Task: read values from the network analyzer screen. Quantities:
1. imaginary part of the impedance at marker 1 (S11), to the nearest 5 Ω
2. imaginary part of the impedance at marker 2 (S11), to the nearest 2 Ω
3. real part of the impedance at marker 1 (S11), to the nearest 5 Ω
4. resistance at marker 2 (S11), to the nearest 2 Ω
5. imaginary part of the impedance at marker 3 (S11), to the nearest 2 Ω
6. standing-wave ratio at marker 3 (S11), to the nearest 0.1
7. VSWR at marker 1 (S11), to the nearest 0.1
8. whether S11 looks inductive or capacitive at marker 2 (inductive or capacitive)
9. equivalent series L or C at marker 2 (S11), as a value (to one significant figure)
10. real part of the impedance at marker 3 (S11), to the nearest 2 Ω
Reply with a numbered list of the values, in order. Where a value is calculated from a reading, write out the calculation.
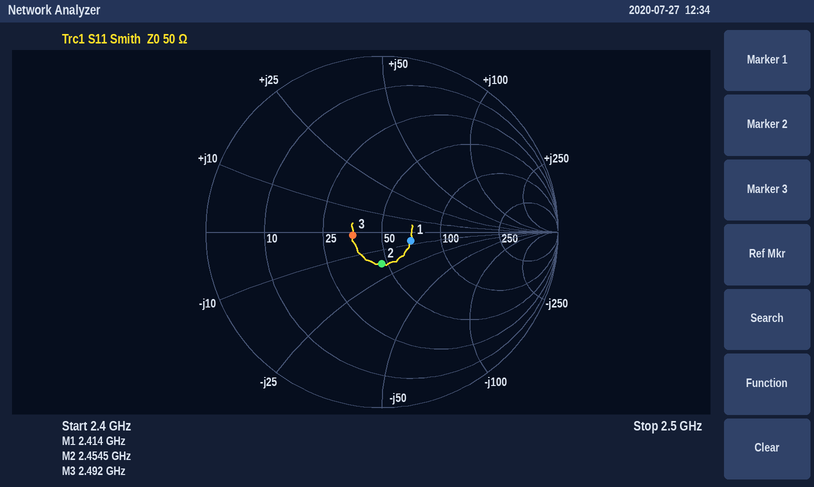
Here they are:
1. -5 Ω
2. -18 Ω
3. 70 Ω
4. 46 Ω
5. -2 Ω
6. 1.4
7. 1.4
8. capacitive
9. C = 1/(2π × 2.4545 GHz × 18 Ω) ≈ 4 pF
10. 36 Ω
